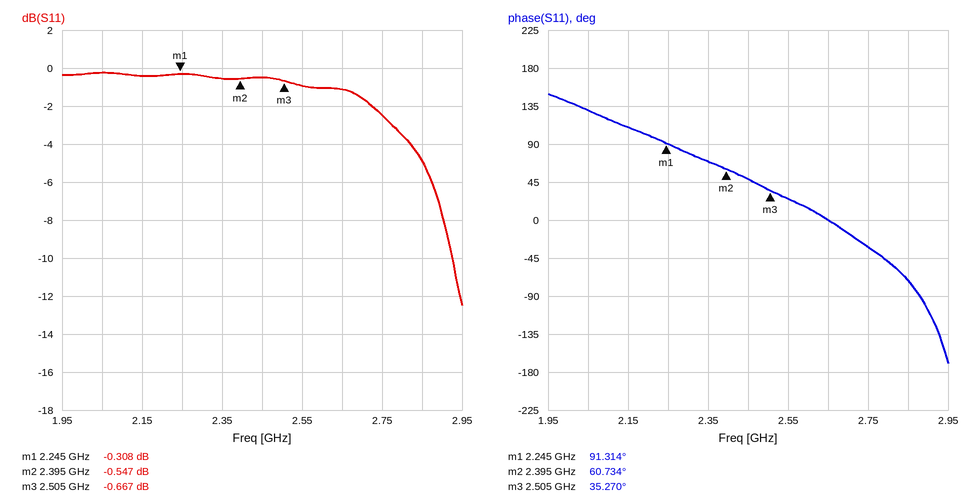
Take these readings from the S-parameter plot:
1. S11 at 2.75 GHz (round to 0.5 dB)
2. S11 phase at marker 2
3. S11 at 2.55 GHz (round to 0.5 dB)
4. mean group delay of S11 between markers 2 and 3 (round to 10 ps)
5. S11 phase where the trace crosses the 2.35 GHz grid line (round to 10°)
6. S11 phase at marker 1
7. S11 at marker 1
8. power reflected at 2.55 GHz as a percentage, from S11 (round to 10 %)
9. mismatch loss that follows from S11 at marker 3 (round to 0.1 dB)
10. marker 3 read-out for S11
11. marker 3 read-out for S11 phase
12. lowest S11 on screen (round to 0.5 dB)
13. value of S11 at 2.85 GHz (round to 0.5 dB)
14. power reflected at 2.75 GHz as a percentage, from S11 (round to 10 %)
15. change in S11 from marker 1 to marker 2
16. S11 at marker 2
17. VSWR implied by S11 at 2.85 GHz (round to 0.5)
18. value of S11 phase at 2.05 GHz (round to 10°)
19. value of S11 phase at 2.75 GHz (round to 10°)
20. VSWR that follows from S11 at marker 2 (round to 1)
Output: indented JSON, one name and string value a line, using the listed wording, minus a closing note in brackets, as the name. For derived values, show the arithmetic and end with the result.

{
  "S11 at 2.75 GHz": "-2.5 dB",
  "S11 phase at marker 2": "60.734°",
  "S11 at 2.55 GHz": "-1.0 dB",
  "mean group delay of S11 between markers 2 and 3": "−(35.27° − (60.734°))/(360° × 110 MHz) ≈ 643 ps, so 640 ps to the nearest 10 ps",
  "S11 phase where the trace crosses the 2.35 GHz grid line": "70°",
  "S11 phase at marker 1": "91.314°",
  "S11 at marker 1": "-0.308 dB",
  "power reflected at 2.55 GHz as a percentage, from S11": "10^(-1/10) ≈ 79.4 %, so 80 % to the nearest 10 %",
  "mismatch loss that follows from S11 at marker 3": "−10 log10(1 − 10^(-0.667/10)) ≈ 8.5 dB",
  "marker 3 read-out for S11": "-0.667 dB",
  "marker 3 read-out for S11 phase": "35.270°",
  "lowest S11 on screen": "-12.5 dB",
  "value of S11 at 2.85 GHz": "-5.0 dB",
  "power reflected at 2.75 GHz as a percentage, from S11": "10^(-2.5/10) ≈ 56.2 %, so 60 % to the nearest 10 %",
  "change in S11 from marker 1 to marker 2": "-0.547 − (-0.308) = -0.239 dB",
  "S11 at marker 2": "-0.547 dB",
  "VSWR implied by S11 at 2.85 GHz": "|Γ| = 10^(-5/20) = 0.5623; VSWR = (1 + 0.5623)/(1 − 0.5623) ≈ 3.57, so 3.5 to the nearest 0.5",
  "value of S11 phase at 2.05 GHz": "130°",
  "value of S11 phase at 2.75 GHz": "-30°",
  "VSWR that follows from S11 at marker 2": "(1 + 0.9390)/(1 − 0.9390) ≈ 32"
}
